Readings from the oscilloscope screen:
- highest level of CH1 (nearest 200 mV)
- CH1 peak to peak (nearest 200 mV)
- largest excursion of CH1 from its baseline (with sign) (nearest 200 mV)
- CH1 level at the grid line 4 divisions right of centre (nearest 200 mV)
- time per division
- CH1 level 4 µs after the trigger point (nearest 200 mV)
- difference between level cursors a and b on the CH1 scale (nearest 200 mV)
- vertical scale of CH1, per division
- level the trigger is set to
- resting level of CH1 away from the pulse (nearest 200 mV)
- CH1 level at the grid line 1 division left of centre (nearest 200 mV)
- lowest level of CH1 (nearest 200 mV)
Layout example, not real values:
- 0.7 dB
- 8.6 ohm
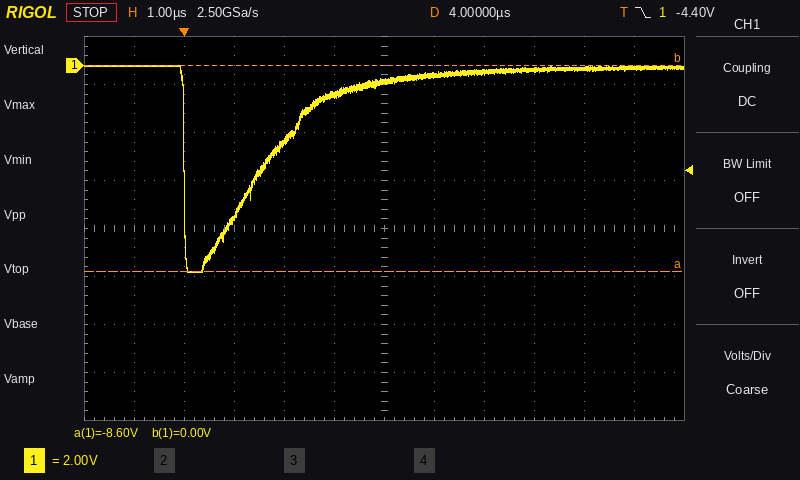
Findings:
- 0.0 V
- 8.6 V
- -8.4 V
- -200 mV
- 1 µs
- -600 mV
- 8.6 V
- 2 V
- -4.40 V
- -200 mV
- -1.2 V
- -8.6 V
